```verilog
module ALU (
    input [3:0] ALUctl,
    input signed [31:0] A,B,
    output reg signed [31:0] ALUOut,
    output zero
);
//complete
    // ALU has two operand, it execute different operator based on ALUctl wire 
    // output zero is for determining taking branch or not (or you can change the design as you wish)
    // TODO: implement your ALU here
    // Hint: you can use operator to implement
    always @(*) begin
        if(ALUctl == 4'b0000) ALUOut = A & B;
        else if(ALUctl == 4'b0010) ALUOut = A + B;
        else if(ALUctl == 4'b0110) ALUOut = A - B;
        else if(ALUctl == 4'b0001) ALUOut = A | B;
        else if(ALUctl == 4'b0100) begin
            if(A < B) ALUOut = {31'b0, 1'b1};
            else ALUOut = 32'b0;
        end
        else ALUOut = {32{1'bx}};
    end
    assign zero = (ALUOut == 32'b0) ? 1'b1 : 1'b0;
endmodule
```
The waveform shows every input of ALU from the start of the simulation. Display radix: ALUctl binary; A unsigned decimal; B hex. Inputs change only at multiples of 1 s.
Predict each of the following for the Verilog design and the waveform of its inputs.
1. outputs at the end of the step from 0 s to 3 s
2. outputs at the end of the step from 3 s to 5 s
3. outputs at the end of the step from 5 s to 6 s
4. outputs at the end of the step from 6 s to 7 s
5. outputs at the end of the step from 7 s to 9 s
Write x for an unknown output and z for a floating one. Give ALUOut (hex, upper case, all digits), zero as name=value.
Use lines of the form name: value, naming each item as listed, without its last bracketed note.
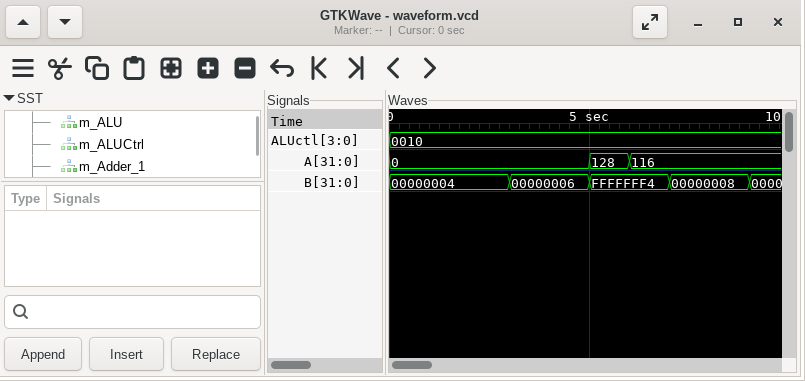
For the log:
outputs at the end of the step from 0 s to 3 s: ALUOut=00000004, zero=0
outputs at the end of the step from 3 s to 5 s: ALUOut=00000006, zero=0
outputs at the end of the step from 5 s to 6 s: ALUOut=00000074, zero=0
outputs at the end of the step from 6 s to 7 s: ALUOut=00000068, zero=0
outputs at the end of the step from 7 s to 9 s: ALUOut=0000007C, zero=0
